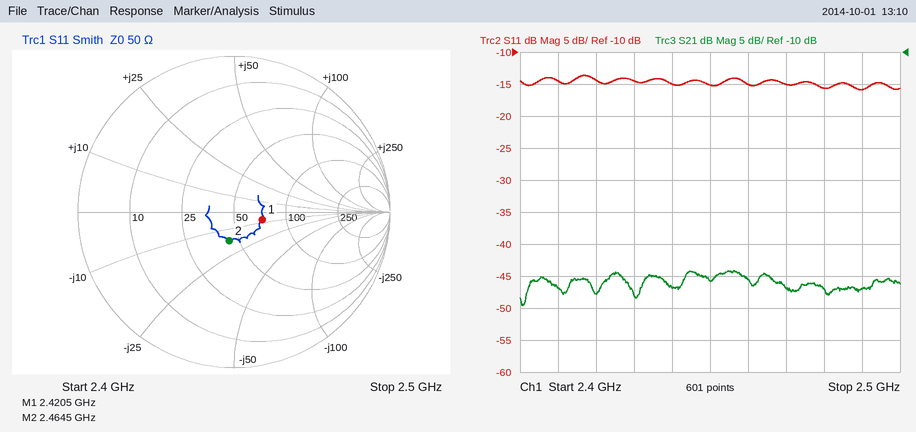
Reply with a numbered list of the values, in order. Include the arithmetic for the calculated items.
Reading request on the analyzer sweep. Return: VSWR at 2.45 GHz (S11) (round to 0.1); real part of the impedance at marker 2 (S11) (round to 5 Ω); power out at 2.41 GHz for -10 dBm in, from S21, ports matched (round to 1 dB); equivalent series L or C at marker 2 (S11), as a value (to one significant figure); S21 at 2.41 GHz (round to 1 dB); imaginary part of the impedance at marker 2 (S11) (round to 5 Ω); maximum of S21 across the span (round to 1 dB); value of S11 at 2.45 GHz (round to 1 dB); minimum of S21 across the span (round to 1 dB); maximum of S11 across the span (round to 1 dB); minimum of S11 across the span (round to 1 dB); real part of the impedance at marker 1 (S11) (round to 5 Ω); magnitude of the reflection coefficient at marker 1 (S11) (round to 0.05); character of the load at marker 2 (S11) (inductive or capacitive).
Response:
1. |Γ| = 10^(-15/20) = 0.1778; VSWR = (1 + 0.1778)/(1 − 0.1778) ≈ 1.4
2. 45 Ω
3. -10 dBm + (-47 dB) = -57 dBm
4. C = 1/(2π × 2.4645 GHz × 15 Ω) ≈ 4 pF
5. -47 dB
6. -15 Ω
7. -44 dB
8. -15 dB
9. -50 dB
10. -14 dB
11. -16 dB
12. 70 Ω
13. 0.20
14. capacitive
